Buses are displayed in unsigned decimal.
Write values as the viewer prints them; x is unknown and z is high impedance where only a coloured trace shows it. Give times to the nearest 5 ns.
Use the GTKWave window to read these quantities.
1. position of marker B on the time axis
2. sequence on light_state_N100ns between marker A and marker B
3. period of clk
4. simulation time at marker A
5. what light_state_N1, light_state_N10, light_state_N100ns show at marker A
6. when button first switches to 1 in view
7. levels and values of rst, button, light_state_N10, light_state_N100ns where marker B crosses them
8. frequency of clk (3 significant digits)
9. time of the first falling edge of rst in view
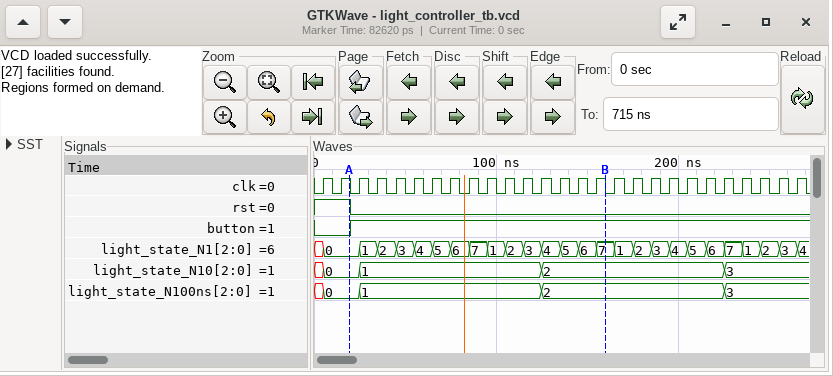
160 ns
0, 1, 2
10 ns
20 ns
light_state_N1=0, light_state_N10=0, light_state_N100ns=0
20 ns
rst=0, button=1, light_state_N10=2, light_state_N100ns=2
100 MHz
20 ns
